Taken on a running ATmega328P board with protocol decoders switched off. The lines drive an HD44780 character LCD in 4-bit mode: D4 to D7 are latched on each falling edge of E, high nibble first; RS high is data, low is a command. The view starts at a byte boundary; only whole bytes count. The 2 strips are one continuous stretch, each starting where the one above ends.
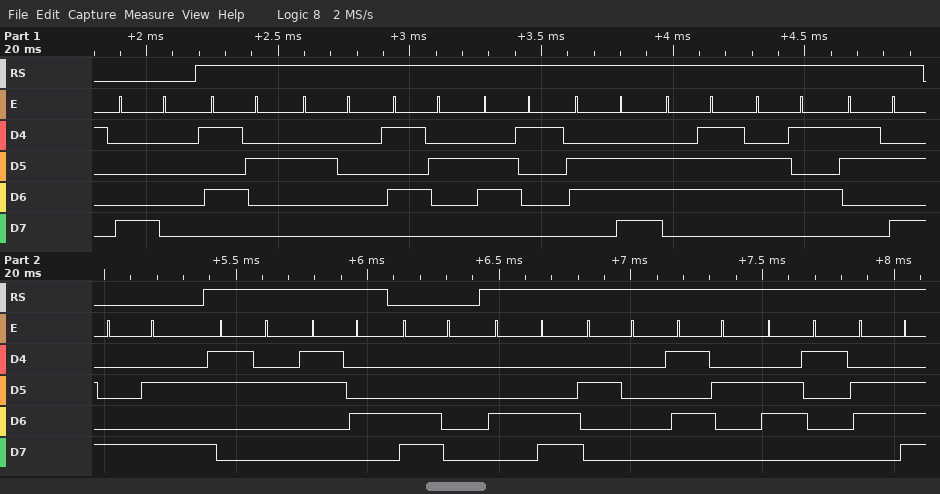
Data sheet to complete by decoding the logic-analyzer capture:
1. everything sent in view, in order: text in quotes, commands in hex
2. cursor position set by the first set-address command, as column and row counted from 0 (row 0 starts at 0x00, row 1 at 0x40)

0x80 "R Range:" 0x8A "24" 0xC0 "L Ran"
column 0, row 0
